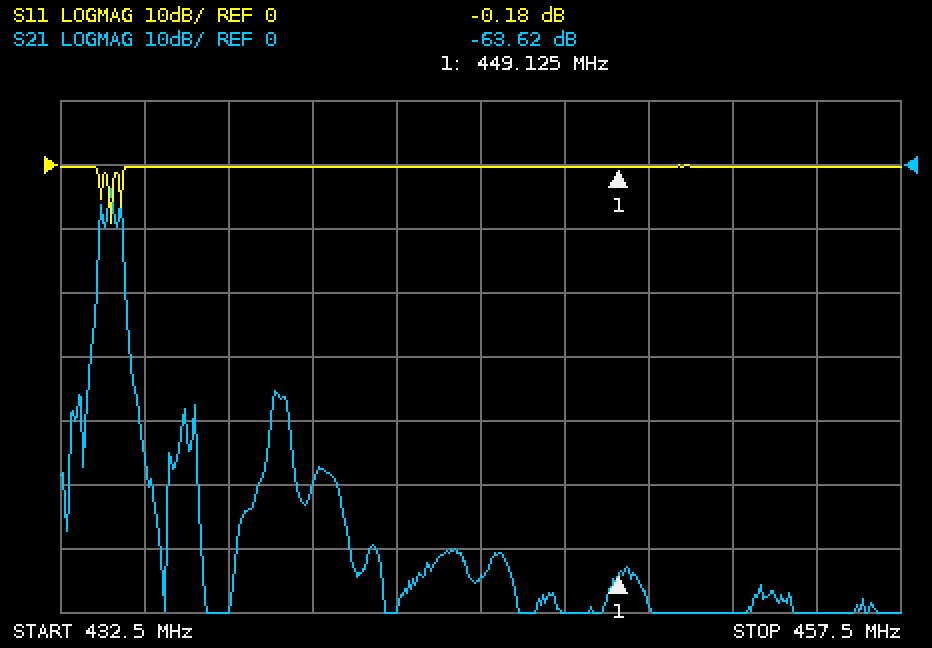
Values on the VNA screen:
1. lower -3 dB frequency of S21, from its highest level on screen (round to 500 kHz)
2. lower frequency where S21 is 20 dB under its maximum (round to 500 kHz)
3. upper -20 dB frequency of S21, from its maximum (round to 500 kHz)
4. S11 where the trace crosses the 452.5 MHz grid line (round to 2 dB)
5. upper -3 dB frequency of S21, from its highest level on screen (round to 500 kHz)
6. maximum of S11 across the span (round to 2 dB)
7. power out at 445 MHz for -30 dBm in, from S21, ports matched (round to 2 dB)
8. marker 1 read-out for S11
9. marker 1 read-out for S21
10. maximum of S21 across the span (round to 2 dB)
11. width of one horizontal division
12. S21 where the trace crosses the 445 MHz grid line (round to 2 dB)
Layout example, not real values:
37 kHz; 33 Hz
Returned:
434.0 MHz; 433.5 MHz; 434.5 MHz; 0 dB; 434.0 MHz; 0 dB; -94 dBm; -0.18 dB; -63.62 dB; -4 dB; 2.5 MHz; -64 dB
